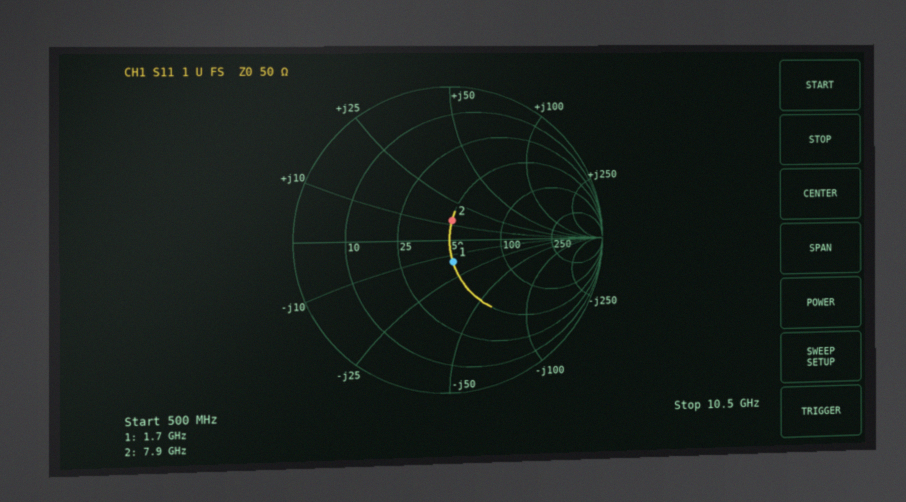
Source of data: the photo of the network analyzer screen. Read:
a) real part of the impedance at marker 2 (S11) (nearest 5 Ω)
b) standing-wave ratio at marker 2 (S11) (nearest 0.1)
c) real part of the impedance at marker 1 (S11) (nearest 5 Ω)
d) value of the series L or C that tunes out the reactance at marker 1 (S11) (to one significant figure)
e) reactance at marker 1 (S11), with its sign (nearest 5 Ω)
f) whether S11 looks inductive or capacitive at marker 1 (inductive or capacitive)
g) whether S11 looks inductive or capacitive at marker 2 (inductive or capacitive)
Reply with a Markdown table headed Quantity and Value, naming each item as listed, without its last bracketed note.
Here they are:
| Quantity | Value |
|---|---|
| real part of the impedance at marker 2 (S11) | 50 Ω |
| standing-wave ratio at marker 2 (S11) | 1.3 |
| real part of the impedance at marker 1 (S11) | 50 Ω |
| value of the series L or C that tunes out the reactance at marker 1 (S11) | 1 nH |
| reactance at marker 1 (S11), with its sign | -15 Ω |
| whether S11 looks inductive or capacitive at marker 1 | capacitive |
| whether S11 looks inductive or capacitive at marker 2 | inductive |
